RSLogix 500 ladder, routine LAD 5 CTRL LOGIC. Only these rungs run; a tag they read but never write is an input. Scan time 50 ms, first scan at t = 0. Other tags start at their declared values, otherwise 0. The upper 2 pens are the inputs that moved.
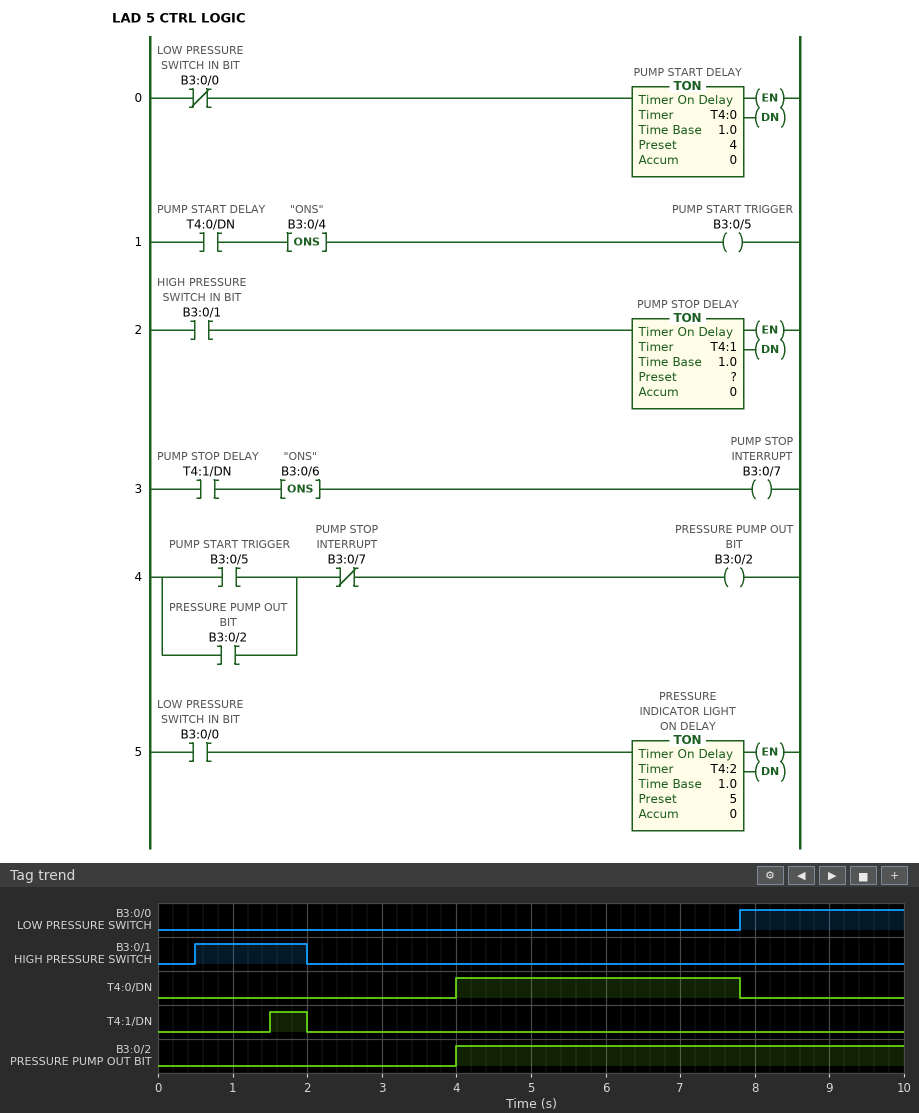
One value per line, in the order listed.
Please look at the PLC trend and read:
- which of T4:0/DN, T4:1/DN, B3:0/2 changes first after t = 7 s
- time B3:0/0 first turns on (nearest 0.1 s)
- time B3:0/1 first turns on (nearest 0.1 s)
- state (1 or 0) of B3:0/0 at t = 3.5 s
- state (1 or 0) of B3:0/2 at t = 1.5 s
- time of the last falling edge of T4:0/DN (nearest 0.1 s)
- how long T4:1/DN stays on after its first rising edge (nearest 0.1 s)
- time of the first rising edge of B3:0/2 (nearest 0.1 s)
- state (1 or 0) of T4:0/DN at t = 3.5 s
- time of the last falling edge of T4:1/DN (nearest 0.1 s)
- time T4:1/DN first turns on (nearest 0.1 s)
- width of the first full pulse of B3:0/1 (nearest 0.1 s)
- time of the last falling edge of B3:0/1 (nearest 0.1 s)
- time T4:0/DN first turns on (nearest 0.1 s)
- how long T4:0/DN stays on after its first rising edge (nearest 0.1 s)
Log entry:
T4:0/DN
7.8 s
0.5 s
0
0
7.8 s
0.5 s
4.0 s
0
2.0 s
1.5 s
1.5 s
2.0 s
4.0 s
3.8 s
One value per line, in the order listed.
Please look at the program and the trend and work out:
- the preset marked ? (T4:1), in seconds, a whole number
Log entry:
1 s
